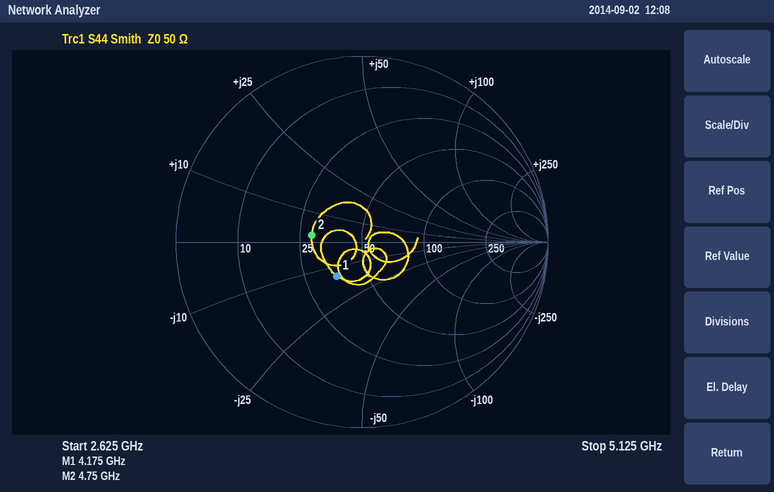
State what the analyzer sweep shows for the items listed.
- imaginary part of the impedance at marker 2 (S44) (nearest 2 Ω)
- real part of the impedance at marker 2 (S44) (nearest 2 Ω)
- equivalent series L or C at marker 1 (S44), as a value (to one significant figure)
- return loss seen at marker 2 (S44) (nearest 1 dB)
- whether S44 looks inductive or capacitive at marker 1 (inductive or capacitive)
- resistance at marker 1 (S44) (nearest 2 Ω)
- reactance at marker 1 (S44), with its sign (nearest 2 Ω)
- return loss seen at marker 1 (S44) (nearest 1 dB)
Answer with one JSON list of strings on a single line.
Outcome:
["+2 Ω", "28 Ω", "3 pF", "11 dB", "capacitive", "36 Ω", "-14 Ω", "13 dB"]
